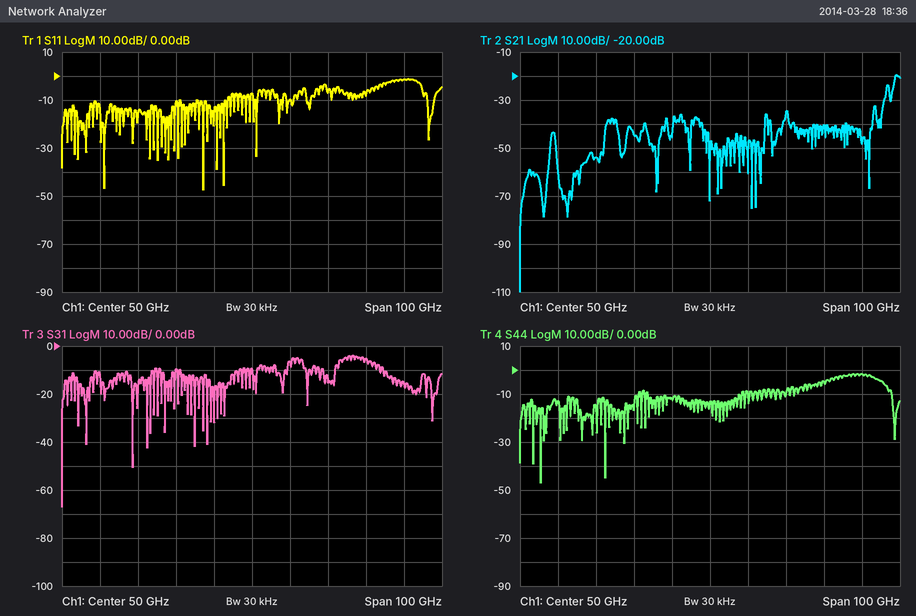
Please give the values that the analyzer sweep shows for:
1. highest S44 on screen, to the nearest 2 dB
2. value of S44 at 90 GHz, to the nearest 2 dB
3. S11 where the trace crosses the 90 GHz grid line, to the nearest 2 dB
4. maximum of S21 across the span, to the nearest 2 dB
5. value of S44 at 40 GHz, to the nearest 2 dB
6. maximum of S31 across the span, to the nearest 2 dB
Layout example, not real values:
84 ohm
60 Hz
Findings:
-2 dB
-2 dB
-2 dB
-20 dB
-12 dB
-4 dB
